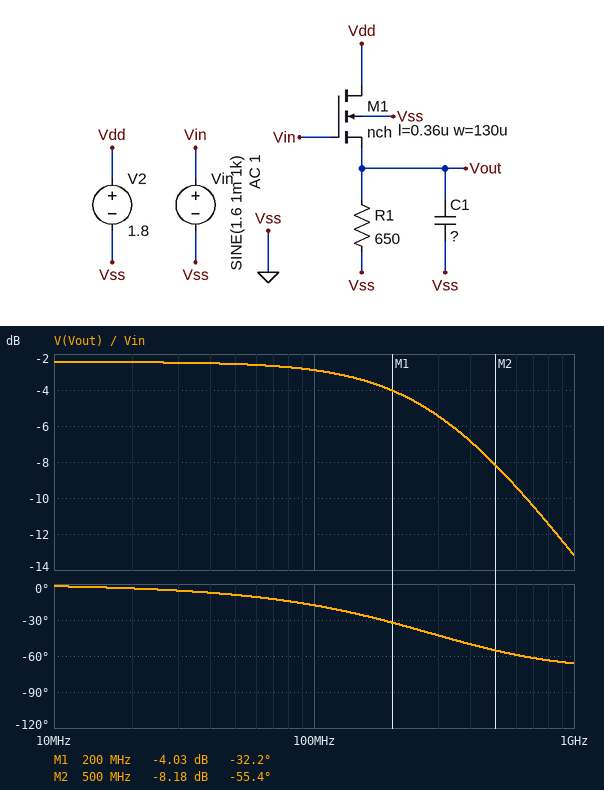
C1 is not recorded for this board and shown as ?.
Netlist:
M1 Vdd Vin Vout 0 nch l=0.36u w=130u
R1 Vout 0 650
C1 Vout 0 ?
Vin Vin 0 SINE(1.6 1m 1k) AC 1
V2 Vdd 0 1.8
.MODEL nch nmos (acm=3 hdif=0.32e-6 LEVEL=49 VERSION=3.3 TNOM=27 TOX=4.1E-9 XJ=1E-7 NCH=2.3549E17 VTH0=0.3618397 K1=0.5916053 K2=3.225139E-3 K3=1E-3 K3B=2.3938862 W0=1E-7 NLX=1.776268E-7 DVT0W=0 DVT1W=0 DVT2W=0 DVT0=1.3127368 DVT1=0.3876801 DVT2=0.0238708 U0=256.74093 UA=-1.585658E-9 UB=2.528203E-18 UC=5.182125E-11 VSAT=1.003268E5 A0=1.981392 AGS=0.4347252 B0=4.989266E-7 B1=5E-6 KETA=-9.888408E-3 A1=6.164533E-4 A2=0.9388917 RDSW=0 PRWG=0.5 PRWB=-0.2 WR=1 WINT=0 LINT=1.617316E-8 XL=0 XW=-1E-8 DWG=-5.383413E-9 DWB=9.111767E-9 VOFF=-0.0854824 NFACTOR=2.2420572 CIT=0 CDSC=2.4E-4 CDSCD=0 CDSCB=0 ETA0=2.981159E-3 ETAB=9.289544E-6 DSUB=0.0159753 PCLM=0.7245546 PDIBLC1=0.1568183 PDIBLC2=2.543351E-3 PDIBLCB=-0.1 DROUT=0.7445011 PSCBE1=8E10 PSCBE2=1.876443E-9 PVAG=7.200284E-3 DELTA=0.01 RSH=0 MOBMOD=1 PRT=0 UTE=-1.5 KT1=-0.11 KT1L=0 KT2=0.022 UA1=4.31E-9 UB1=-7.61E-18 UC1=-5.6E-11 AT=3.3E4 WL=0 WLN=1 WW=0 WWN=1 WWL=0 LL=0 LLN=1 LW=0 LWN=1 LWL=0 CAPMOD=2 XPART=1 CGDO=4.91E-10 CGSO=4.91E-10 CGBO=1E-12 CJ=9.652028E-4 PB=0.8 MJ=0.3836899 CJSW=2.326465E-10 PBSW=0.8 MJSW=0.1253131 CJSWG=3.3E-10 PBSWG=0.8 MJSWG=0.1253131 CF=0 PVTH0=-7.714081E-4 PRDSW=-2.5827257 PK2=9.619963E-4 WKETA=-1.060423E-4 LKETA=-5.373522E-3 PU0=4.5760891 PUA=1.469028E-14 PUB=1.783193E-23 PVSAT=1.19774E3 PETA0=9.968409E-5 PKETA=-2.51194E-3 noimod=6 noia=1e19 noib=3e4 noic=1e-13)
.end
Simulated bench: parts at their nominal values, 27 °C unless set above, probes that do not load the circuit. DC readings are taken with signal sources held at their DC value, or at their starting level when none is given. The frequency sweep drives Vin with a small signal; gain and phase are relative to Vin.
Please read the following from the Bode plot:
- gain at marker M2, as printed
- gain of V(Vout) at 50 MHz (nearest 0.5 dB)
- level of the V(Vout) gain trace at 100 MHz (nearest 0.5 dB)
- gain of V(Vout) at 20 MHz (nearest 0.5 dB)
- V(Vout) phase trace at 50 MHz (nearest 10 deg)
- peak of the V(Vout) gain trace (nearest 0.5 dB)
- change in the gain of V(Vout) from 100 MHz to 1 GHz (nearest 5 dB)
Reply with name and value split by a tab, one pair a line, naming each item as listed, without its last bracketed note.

gain at marker M2, as printed	-8.18 dB
gain of V(Vout) at 50 MHz	-2.5 dB
level of the V(Vout) gain trace at 100 MHz	-3.0 dB
gain of V(Vout) at 20 MHz	-2.5 dB
V(Vout) phase trace at 50 MHz	-10 deg
peak of the V(Vout) gain trace	-2.5 dB
change in the gain of V(Vout) from 100 MHz to 1 GHz	-10 dB
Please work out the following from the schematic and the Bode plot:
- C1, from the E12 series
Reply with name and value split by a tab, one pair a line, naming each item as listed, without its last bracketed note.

C1, from the E12 series	10 pF
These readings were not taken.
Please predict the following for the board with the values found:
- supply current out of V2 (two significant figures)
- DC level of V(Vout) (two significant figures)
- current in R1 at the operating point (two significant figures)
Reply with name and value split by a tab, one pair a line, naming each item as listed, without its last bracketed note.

supply current out of V2	1.2 mA
DC level of V(Vout)	790 mV
current in R1 at the operating point	1.2 mA
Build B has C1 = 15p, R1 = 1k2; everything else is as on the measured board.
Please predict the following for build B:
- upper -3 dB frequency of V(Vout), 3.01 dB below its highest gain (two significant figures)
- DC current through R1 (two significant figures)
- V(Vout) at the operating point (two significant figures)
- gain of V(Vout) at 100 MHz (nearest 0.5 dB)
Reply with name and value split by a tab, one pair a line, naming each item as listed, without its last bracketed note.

upper -3 dB frequency of V(Vout), 3.01 dB below its highest gain	140 MHz
DC current through R1	690 µA
V(Vout) at the operating point	830 mV
gain of V(Vout) at 100 MHz	-4.0 dB
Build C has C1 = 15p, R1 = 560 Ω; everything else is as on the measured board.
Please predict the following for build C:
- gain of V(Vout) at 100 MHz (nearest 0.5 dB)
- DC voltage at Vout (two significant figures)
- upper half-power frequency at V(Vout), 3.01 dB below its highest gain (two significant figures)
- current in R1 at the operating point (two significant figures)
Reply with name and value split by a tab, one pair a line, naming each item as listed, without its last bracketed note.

gain of V(Vout) at 100 MHz	-3.5 dB
DC voltage at Vout	780 mV
upper half-power frequency at V(Vout), 3.01 dB below its highest gain	220 MHz
current in R1 at the operating point	1.4 mA
